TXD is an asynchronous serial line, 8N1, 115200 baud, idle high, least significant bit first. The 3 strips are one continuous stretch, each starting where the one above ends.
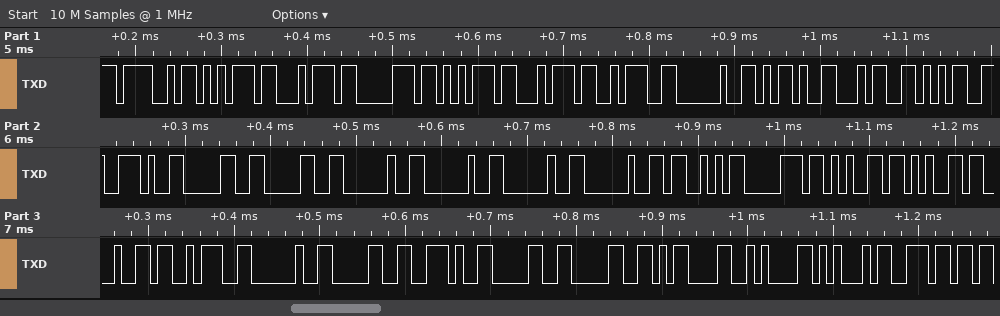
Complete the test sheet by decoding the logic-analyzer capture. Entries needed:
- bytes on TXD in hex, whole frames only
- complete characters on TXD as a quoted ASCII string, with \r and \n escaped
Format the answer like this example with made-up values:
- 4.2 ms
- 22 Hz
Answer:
- 4F 75 74 70 75 74 3A 20 2D 34 35 2E 30 30 20 20 20 20 53 70 65 65 64 3A 20 30 2E 30 30 0D 0A 45 6E
- "Output: -45.00    Speed: 0.00\r\nEn"
